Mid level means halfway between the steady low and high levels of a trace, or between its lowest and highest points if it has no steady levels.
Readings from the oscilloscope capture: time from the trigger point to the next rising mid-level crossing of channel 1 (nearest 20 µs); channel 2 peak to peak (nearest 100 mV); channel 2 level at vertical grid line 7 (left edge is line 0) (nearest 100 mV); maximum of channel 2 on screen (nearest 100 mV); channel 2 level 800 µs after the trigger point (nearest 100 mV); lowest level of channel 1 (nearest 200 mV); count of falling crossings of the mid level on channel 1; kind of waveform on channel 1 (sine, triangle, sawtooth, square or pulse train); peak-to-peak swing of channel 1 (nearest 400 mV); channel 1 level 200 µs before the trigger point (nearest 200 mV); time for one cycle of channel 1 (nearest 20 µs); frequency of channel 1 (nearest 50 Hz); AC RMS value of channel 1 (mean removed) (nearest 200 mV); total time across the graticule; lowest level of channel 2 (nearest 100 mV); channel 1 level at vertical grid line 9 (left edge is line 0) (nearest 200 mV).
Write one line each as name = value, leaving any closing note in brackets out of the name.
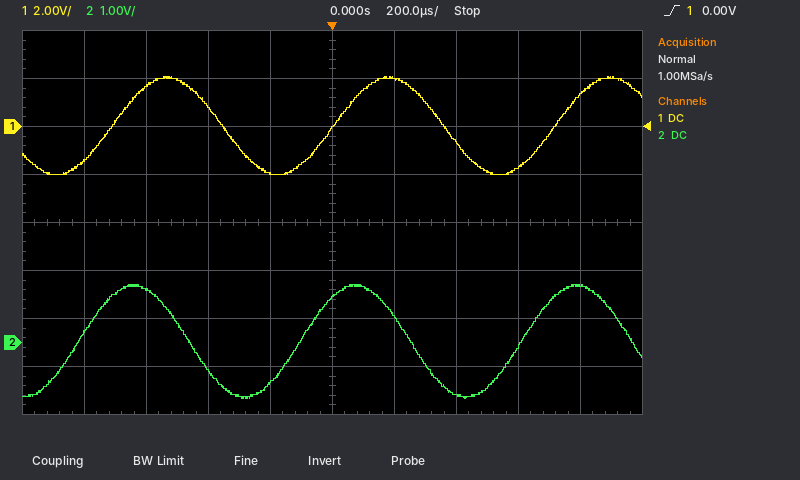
time from the trigger point to the next rising mid-level crossing of channel 1 = 720 µs
channel 2 peak to peak = 2.4 V
channel 2 level at vertical grid line 7 (left edge is line 0) = -1.1 V
maximum of channel 2 on screen = 1.2 V
channel 2 level 800 µs after the trigger point = 1.2 V
lowest level of channel 1 = -2.0 V
count of falling crossings of the mid level on channel 1 = 2
kind of waveform on channel 1 = sine
peak-to-peak swing of channel 1 = 4.0 V
channel 1 level 200 µs before the trigger point = -2.0 V
time for one cycle of channel 1 = 720 µs
frequency of channel 1 = 1.40 kHz
AC RMS value of channel 1 (mean removed) = 1.4 V
total time across the graticule = 2 ms
lowest level of channel 2 = -1.2 V
channel 1 level at vertical grid line 9 (left edge is line 0) = 1.4 V
